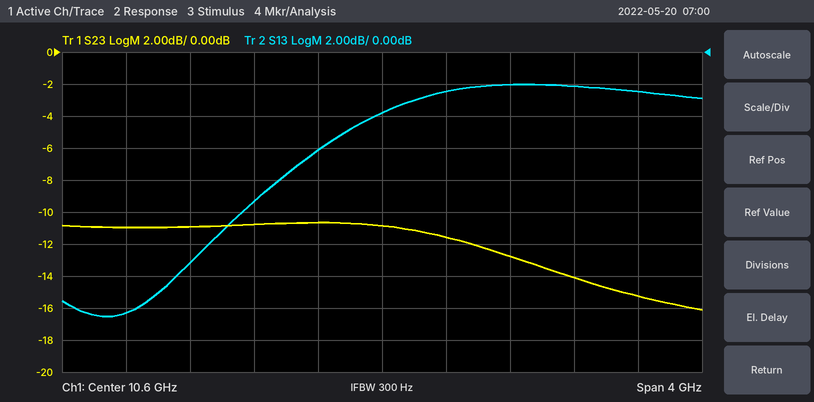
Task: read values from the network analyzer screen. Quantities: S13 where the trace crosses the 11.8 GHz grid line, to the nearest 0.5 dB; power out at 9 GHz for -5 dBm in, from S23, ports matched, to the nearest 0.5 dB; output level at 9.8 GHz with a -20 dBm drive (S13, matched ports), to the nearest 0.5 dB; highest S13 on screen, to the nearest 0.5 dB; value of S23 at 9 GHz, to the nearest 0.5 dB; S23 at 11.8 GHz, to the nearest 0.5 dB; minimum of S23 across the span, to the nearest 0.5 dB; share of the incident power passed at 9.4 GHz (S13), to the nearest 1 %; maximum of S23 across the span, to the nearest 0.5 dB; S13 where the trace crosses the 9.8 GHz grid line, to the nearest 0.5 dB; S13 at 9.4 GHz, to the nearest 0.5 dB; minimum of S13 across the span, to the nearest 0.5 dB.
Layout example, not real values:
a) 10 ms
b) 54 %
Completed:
a) -2.0 dB
b) -16.0 dBm
c) -29.5 dBm
d) -2.0 dB
e) -11.0 dB
f) -14.0 dB
g) -16.0 dB
h) 5 %
i) -10.5 dB
j) -9.5 dB
k) -13.0 dB
l) -16.5 dB
